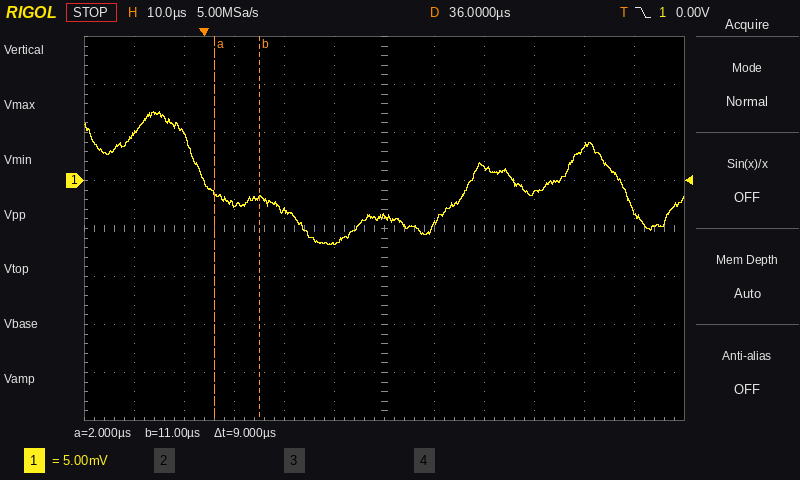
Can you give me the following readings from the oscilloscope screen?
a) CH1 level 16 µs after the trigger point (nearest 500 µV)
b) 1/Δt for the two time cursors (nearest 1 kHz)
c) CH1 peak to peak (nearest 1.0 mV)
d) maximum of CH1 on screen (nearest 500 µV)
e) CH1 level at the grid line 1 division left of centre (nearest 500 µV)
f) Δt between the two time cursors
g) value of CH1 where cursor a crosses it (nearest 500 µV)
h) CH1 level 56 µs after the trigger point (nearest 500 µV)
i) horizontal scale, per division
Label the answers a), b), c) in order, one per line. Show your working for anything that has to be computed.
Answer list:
a) -3.0 mV
b) 1 / 9 µs ≈ 111 kHz
c) 14.0 mV
d) 7.0 mV
e) -6.5 mV
f) 9 µs
g) -1.5 mV
h) 1.5 mV
i) 10 µs
